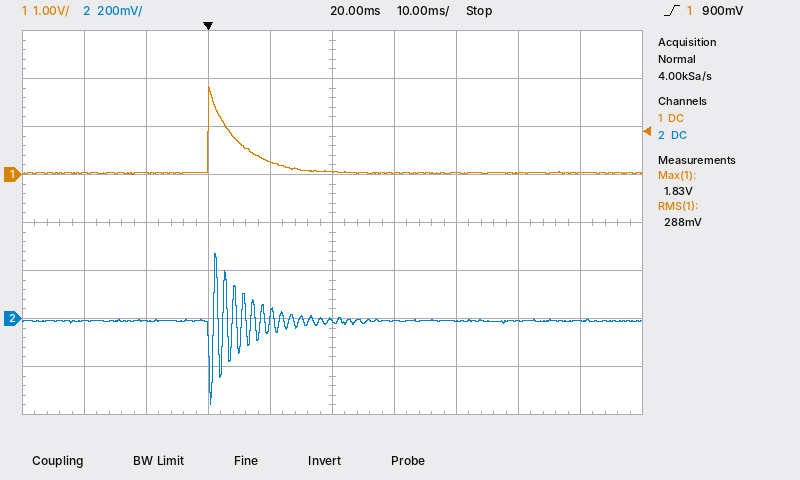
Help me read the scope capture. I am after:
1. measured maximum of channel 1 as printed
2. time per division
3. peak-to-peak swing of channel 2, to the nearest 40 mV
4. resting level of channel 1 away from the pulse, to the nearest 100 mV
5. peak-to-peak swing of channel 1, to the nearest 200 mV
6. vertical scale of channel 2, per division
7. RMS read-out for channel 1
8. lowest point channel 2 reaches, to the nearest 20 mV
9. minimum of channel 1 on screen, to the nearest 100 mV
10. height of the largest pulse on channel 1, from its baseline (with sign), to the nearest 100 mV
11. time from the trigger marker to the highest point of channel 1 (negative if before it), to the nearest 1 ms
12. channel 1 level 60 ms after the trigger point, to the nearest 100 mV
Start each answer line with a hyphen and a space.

- 1.83 V
- 10 ms
- 640 mV
- 0.0 V
- 1.8 V
- 200 mV
- 288 mV
- -360 mV
- 0.0 V
- +1.8 V
- 0 ms
- 0.0 V
